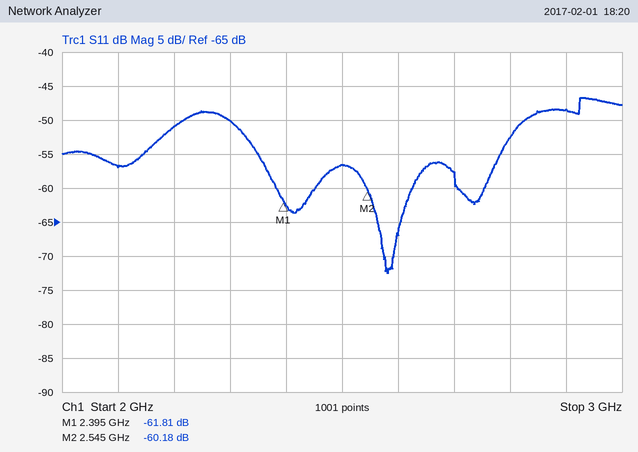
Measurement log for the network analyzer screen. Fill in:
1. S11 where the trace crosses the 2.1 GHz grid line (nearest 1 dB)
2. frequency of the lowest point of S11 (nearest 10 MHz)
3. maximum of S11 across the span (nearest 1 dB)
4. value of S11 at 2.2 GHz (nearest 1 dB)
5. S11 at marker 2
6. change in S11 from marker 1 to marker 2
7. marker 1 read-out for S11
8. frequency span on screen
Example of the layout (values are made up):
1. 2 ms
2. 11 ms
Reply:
1. -57 dB
2. 2.58 GHz
3. -47 dB
4. -51 dB
5. -60.18 dB
6. 1.63 dB
7. -61.81 dB
8. 1 GHz
